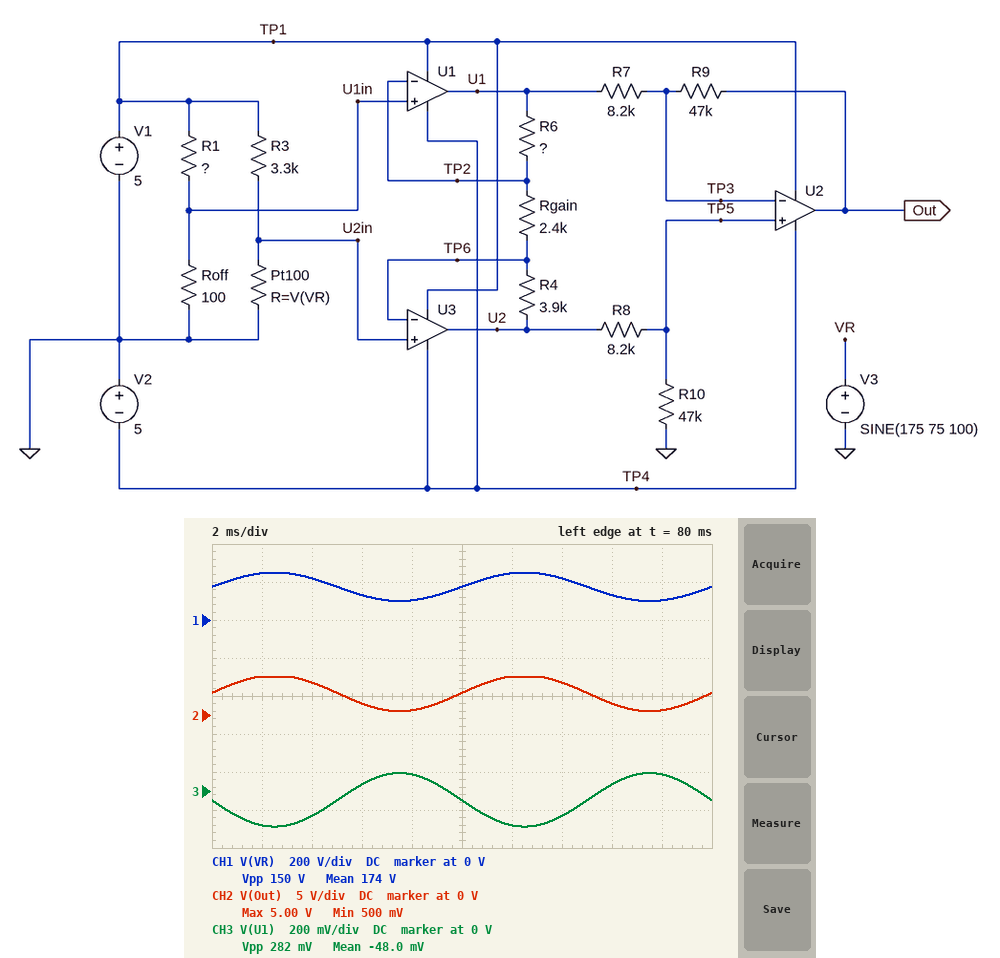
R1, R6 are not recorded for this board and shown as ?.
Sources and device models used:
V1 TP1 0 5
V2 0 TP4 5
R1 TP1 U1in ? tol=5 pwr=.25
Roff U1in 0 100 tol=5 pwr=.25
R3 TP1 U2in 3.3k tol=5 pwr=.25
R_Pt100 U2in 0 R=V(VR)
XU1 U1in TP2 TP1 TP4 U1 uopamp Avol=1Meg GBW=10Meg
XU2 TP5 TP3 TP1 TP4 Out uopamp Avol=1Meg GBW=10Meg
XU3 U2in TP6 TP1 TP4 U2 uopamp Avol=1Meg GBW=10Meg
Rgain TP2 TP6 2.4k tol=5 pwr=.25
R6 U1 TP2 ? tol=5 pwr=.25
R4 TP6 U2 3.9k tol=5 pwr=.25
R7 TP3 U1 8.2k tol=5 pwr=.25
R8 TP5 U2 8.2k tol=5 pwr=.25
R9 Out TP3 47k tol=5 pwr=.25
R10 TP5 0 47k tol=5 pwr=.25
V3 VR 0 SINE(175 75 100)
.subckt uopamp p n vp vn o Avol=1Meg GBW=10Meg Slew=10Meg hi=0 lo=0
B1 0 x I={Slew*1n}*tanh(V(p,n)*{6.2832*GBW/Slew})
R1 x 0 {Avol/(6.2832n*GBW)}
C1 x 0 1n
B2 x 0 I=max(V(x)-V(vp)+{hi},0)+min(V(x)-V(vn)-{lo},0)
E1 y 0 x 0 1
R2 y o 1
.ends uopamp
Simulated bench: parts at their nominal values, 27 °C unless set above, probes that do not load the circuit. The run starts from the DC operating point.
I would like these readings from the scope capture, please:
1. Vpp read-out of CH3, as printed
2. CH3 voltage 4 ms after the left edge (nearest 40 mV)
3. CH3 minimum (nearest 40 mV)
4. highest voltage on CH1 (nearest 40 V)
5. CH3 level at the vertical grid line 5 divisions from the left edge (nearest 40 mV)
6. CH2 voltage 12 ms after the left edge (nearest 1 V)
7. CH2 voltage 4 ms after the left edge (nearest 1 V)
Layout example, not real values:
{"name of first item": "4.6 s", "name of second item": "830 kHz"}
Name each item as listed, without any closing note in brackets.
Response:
{"Vpp read-out of CH3, as printed": "282 mV", "CH3 voltage 4 ms after the left edge": "-120 mV", "CH3 minimum": "-200 mV", "highest voltage on CH1": "240 V", "CH3 level at the vertical grid line 5 divisions from the left edge": "-40 mV", "CH2 voltage 12 ms after the left edge": "5 V", "CH2 voltage 4 ms after the left edge": "4 V"}
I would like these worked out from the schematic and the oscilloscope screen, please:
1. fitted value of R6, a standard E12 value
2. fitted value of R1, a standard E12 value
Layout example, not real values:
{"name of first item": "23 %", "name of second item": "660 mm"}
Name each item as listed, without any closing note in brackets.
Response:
{"fitted value of R6, a standard E12 value": "3.3 kΩ", "fitted value of R1, a standard E12 value": "3.9 kΩ"}
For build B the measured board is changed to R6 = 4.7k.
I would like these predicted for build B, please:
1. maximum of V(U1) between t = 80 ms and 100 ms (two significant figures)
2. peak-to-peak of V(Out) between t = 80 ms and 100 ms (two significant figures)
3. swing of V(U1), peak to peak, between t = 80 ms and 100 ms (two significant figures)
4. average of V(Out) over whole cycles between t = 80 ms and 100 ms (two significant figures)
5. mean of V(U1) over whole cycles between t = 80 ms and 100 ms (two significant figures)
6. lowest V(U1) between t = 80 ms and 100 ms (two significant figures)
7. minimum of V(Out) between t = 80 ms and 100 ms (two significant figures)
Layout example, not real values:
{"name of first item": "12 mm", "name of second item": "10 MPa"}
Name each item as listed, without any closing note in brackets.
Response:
{"maximum of V(U1) between t = 80 ms and 100 ms": "82 mV", "peak-to-peak of V(Out) between t = 80 ms and 100 ms": "4.4 V", "swing of V(U1), peak to peak, between t = 80 ms and 100 ms": "400 mV", "average of V(Out) over whole cycles between t = 80 ms and 100 ms": "3.1 V", "mean of V(U1) over whole cycles between t = 80 ms and 100 ms": "-120 mV", "lowest V(U1) between t = 80 ms and 100 ms": "-320 mV", "minimum of V(Out) between t = 80 ms and 100 ms": "580 mV"}
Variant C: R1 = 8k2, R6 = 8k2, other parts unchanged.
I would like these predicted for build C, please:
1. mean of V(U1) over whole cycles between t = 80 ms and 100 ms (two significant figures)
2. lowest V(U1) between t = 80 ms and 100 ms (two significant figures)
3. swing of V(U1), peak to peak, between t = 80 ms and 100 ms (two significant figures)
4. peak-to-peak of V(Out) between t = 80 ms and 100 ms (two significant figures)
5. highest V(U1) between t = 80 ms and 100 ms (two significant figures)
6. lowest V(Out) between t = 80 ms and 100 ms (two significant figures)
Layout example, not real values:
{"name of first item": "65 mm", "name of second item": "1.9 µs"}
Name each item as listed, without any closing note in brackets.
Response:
{"mean of V(U1) over whole cycles between t = 80 ms and 100 ms": "-590 mV", "lowest V(U1) between t = 80 ms and 100 ms": "-940 mV", "swing of V(U1), peak to peak, between t = 80 ms and 100 ms": "700 mV", "peak-to-peak of V(Out) between t = 80 ms and 100 ms": "2.0 V", "highest V(U1) between t = 80 ms and 100 ms": "-240 mV", "lowest V(Out) between t = 80 ms and 100 ms": "3.0 V"}
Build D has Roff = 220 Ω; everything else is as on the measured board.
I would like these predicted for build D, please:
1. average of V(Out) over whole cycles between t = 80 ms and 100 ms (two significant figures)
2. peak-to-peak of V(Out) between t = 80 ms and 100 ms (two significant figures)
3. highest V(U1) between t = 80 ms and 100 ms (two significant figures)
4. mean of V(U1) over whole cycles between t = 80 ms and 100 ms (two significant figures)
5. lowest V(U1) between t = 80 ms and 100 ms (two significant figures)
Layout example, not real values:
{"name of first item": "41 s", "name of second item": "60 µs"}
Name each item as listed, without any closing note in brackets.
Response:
{"average of V(Out) over whole cycles between t = 80 ms and 100 ms": "-370 mV", "peak-to-peak of V(Out) between t = 80 ms and 100 ms": "4.7 V", "highest V(U1) between t = 80 ms and 100 ms": "430 mV", "mean of V(U1) over whole cycles between t = 80 ms and 100 ms": "290 mV", "lowest V(U1) between t = 80 ms and 100 ms": "150 mV"}
